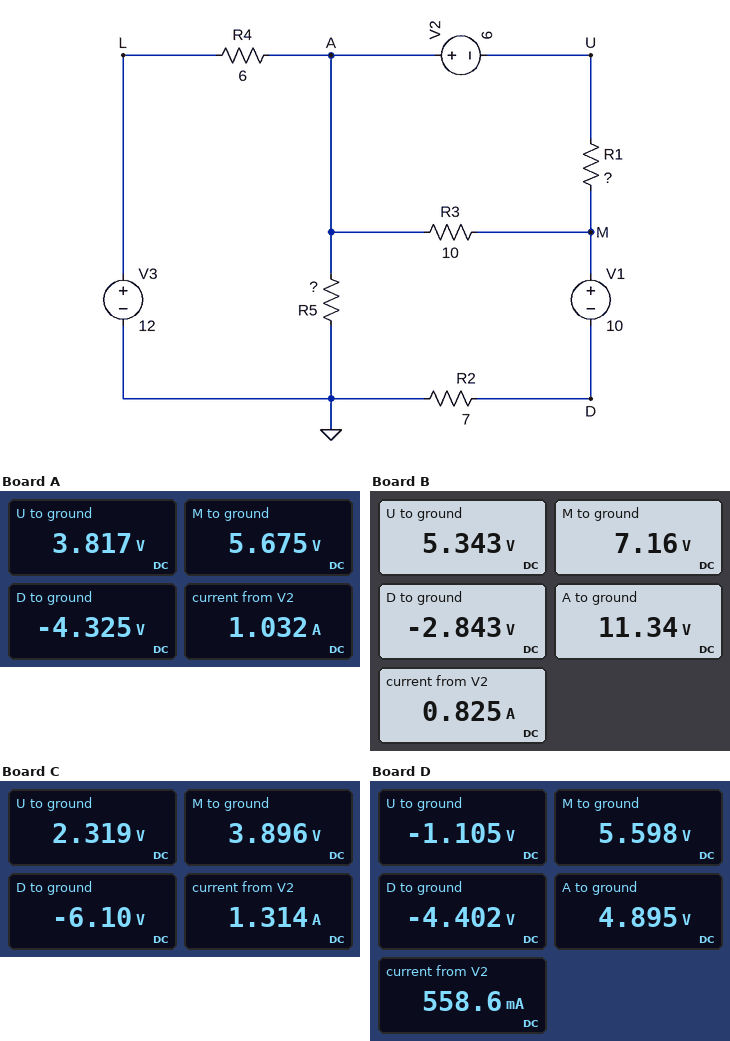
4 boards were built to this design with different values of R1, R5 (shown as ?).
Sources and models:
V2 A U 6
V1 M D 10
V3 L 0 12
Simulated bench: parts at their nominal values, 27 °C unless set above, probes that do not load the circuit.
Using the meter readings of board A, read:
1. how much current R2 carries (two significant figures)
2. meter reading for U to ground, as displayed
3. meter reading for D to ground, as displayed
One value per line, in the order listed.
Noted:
620 mA
3.817 V
-4.325 V
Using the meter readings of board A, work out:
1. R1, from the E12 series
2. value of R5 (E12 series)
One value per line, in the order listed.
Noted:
1.8 Ω
10 Ω
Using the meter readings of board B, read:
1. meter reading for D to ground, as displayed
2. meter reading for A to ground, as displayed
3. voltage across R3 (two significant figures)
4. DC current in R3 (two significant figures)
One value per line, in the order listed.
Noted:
-2.843 V
11.34 V
4.2 V
420 mA
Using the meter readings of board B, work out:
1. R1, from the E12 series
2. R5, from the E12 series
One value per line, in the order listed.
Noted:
2.2 Ω
22 Ω
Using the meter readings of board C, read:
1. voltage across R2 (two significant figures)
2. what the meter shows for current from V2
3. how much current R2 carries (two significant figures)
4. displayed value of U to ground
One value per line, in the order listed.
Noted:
6.1 V
1.314 A
870 mA
2.319 V
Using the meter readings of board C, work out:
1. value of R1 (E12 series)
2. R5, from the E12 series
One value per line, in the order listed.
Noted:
1.2 Ω
5.6 Ω
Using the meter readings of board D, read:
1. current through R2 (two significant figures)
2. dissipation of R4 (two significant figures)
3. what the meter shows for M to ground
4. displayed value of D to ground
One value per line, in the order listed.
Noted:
630 mA
8.4 W
5.598 V
-4.402 V
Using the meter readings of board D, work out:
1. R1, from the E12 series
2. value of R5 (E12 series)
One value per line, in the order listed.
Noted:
12 Ω
2.7 Ω
